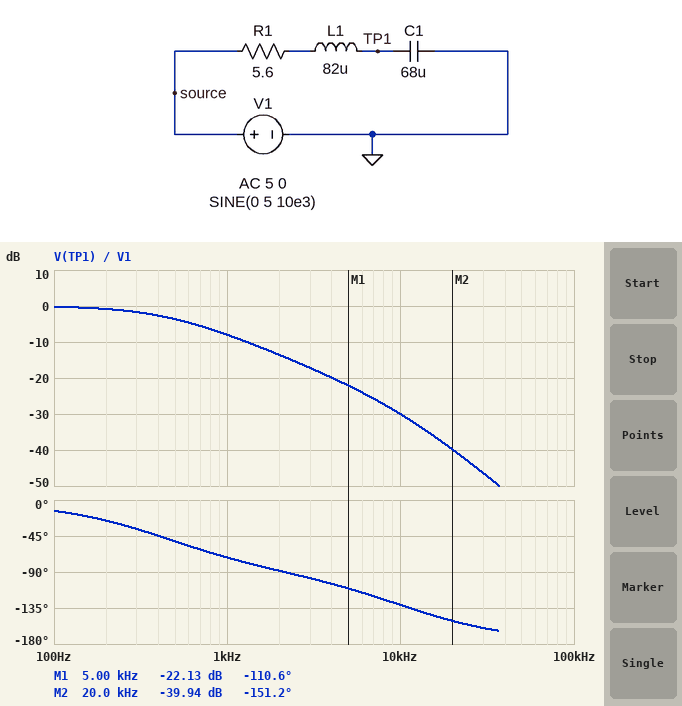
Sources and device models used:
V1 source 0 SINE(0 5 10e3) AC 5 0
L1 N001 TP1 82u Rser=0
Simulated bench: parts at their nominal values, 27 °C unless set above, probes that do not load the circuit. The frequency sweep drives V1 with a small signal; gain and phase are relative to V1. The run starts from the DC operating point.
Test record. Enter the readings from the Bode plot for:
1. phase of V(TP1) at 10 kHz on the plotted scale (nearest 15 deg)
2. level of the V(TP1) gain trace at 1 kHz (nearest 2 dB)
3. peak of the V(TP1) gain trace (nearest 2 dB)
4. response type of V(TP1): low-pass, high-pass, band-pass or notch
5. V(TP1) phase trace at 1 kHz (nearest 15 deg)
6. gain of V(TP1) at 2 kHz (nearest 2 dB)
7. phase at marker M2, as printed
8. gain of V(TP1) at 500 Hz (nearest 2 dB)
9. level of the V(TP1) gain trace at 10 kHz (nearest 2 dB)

-135 deg
-8 dB
0 dB
low-pass
-75 deg
-14 dB
-151.2 deg
-4 dB
-30 dB
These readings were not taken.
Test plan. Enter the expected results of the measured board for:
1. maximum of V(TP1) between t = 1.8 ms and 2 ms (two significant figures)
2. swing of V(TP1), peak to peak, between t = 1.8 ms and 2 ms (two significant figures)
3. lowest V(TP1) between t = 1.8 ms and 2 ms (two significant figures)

160 mV
310 mV
-160 mV
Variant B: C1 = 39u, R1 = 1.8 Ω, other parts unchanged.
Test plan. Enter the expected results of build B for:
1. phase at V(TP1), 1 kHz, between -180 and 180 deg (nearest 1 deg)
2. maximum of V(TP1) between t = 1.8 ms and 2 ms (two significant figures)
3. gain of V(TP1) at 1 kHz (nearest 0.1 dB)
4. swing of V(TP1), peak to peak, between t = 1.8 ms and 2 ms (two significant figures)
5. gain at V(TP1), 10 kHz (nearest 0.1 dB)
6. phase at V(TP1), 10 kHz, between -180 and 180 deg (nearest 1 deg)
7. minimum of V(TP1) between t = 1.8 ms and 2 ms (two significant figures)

-27 deg
400 mV
0.2 dB
800 mV
-21.9 dB
-159 deg
-400 mV
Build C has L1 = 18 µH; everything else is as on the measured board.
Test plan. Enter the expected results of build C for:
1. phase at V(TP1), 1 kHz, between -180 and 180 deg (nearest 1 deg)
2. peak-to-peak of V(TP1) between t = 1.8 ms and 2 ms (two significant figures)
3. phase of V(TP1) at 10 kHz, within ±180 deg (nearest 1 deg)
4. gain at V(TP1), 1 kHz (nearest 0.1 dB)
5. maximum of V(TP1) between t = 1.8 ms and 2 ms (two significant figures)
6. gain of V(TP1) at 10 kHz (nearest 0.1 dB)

-68 deg
410 mV
-99 deg
-8.2 dB
210 mV
-27.7 dB
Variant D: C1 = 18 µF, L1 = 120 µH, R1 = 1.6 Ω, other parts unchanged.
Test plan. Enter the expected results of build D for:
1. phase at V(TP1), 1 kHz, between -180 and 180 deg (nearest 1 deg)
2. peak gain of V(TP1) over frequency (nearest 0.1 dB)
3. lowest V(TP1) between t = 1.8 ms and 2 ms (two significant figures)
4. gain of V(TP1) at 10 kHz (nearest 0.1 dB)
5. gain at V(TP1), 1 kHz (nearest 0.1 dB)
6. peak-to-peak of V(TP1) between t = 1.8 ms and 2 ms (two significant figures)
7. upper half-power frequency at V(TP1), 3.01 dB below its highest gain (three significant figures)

-11 deg
4.6 dB
-650 mV
-17.8 dB
0.6 dB
1.3 V
4.05 kHz
